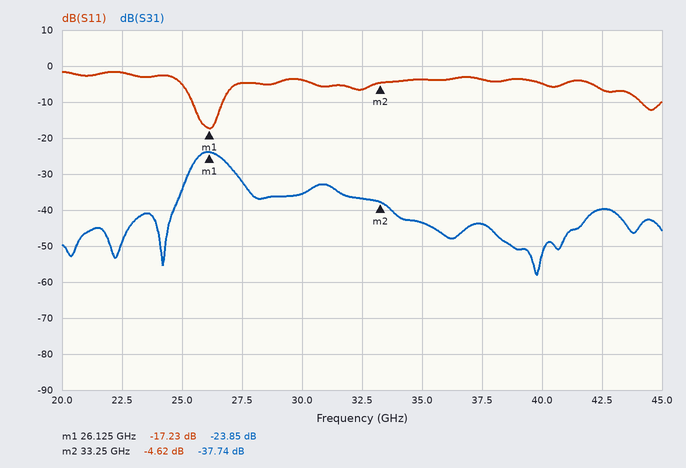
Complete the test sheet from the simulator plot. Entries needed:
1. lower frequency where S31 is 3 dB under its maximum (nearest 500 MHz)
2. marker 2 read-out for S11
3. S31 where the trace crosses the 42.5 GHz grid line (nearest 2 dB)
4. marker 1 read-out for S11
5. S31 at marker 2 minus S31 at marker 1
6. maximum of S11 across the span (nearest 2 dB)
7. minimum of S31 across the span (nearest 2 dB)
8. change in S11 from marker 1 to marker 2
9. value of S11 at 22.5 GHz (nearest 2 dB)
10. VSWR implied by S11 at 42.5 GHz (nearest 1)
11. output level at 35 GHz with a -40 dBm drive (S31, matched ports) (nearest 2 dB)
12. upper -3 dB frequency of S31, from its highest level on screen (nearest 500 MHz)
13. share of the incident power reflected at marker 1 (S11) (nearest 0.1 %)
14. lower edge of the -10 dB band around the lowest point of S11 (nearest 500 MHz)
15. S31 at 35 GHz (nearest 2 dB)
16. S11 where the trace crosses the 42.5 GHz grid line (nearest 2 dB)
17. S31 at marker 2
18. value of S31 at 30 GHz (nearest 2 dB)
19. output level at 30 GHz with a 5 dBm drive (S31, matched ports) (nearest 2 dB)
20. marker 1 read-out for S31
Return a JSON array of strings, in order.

["25.5 GHz", "-4.62 dB", "-40 dB", "-17.23 dB", "-13.89 dB", "-2 dB", "-58 dB", "12.61 dB", "-2 dB", "3", "-84 dBm", "27.0 GHz", "1.9 %", "25.5 GHz", "-44 dB", "-6 dB", "-37.74 dB", "-36 dB", "-30 dBm", "-23.85 dB"]
